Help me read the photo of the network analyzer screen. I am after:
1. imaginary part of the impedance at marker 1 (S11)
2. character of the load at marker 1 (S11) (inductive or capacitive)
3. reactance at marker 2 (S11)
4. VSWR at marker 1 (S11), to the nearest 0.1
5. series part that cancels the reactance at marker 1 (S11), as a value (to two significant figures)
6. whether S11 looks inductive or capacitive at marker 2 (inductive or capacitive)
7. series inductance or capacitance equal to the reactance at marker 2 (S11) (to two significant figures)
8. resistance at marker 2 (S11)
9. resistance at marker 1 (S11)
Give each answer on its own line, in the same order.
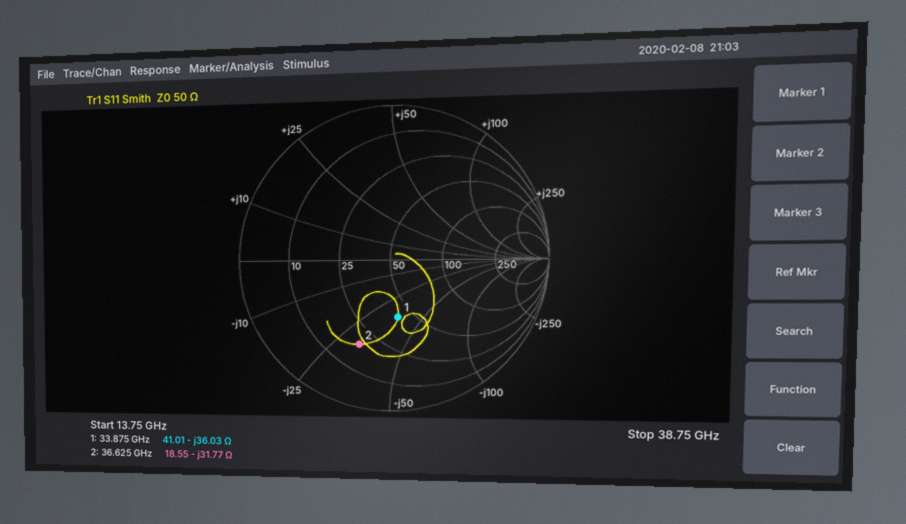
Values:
-36.03 Ω
capacitive
-31.77 Ω
2.2
170 pH
capacitive
140 fF
18.55 Ω
41.01 Ω
